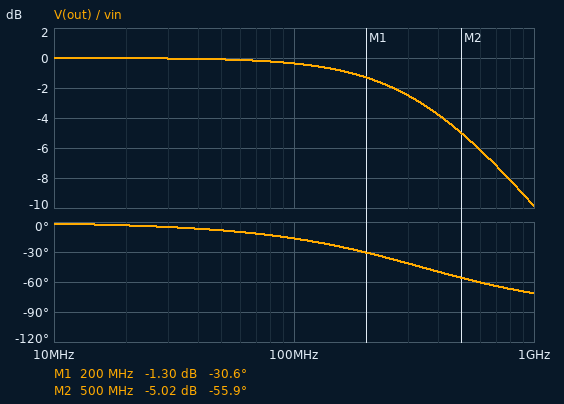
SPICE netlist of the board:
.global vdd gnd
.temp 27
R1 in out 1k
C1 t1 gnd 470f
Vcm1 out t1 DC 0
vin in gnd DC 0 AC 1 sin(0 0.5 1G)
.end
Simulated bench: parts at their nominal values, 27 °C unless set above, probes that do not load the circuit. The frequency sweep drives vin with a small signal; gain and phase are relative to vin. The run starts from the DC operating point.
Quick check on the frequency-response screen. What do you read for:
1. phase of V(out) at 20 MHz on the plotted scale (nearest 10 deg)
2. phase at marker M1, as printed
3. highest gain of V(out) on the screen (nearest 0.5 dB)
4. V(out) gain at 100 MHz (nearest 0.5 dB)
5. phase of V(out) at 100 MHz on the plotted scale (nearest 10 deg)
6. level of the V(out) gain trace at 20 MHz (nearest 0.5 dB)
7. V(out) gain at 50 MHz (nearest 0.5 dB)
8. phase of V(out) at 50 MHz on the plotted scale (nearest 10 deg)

0 deg
-30.6 deg
0 dB
-0.5 dB
-20 deg
0 dB
0 dB
-10 deg
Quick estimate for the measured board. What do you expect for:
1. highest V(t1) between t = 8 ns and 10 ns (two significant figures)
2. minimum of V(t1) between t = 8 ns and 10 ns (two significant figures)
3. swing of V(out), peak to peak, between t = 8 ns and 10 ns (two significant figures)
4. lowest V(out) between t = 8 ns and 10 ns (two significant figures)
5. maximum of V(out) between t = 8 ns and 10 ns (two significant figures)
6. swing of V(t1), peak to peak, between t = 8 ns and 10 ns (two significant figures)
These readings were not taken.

160 mV
-160 mV
320 mV
-160 mV
160 mV
320 mV
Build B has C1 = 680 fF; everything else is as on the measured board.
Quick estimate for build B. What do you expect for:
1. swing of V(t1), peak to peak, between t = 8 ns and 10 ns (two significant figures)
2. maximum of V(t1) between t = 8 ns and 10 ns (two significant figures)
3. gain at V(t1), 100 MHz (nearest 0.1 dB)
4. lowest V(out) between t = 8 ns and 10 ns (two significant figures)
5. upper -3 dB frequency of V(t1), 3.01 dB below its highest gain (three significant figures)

230 mV
110 mV
-0.7 dB
-110 mV
234 MHz
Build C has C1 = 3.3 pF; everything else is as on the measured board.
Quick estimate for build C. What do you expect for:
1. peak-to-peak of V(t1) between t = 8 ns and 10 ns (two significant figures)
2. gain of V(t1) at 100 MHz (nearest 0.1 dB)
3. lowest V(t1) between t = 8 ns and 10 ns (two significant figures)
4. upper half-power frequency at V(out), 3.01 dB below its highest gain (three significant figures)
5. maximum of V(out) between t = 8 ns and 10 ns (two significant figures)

49 mV
-7.2 dB
-23 mV
48.2 MHz
26 mV
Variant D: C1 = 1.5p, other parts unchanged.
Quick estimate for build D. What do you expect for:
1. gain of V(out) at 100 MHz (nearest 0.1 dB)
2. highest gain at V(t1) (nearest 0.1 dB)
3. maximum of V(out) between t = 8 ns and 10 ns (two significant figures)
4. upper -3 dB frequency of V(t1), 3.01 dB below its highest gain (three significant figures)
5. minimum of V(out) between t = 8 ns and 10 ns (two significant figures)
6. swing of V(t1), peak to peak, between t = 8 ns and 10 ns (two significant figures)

-2.8 dB
0 dB
53 mV
106 MHz
-53 mV
110 mV
